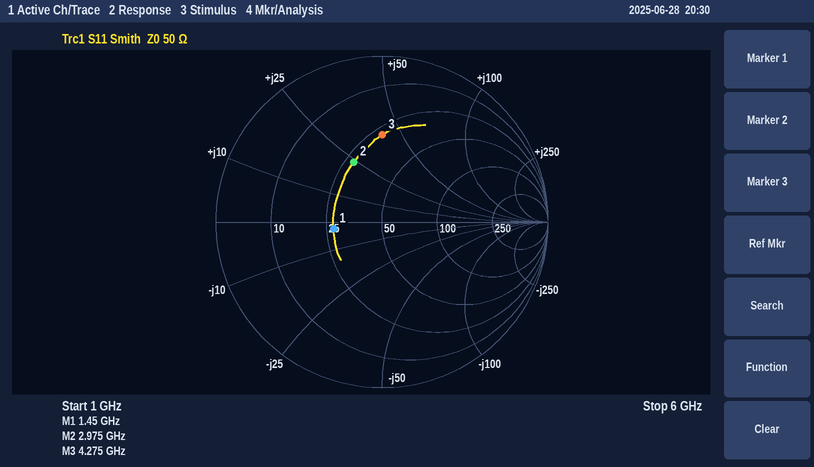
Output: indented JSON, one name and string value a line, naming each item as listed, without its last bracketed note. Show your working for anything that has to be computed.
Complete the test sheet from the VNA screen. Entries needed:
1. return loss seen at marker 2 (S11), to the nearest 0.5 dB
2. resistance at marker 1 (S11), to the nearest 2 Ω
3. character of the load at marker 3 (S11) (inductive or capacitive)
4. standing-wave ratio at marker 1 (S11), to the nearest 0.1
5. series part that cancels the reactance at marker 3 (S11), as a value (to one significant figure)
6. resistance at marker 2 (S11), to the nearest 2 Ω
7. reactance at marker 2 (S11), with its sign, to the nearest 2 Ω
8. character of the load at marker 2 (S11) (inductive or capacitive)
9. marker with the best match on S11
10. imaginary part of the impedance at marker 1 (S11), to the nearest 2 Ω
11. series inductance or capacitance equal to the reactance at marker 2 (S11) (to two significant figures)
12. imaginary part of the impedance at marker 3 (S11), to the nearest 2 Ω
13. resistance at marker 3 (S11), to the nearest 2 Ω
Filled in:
{
  "return loss seen at marker 2 (S11), to the nearest 0.5 dB": "8.0 dB",
  "resistance at marker 1 (S11), to the nearest 2 Ω": "28 Ω",
  "character of the load at marker 3 (S11)": "inductive",
  "standing-wave ratio at marker 1 (S11), to the nearest 0.1": "1.8",
  "series part that cancels the reactance at marker 3 (S11), as a value": "C = 1/(2π × 4.275 GHz × 42 Ω) ≈ 886 fF, so 900 fF to one significant figure",
  "resistance at marker 2 (S11), to the nearest 2 Ω": "28 Ω",
  "reactance at marker 2 (S11), with its sign, to the nearest 2 Ω": "+24 Ω",
  "character of the load at marker 2 (S11)": "inductive",
  "marker with the best match on S11": "marker 1",
  "imaginary part of the impedance at marker 1 (S11), to the nearest 2 Ω": "-2 Ω",
  "series inductance or capacitance equal to the reactance at marker 2 (S11)": "L = 24 Ω/(2π × 2.975 GHz) ≈ 1.3 nH",
  "imaginary part of the impedance at marker 3 (S11), to the nearest 2 Ω": "+42 Ω",
  "resistance at marker 3 (S11), to the nearest 2 Ω": "28 Ω"
}
